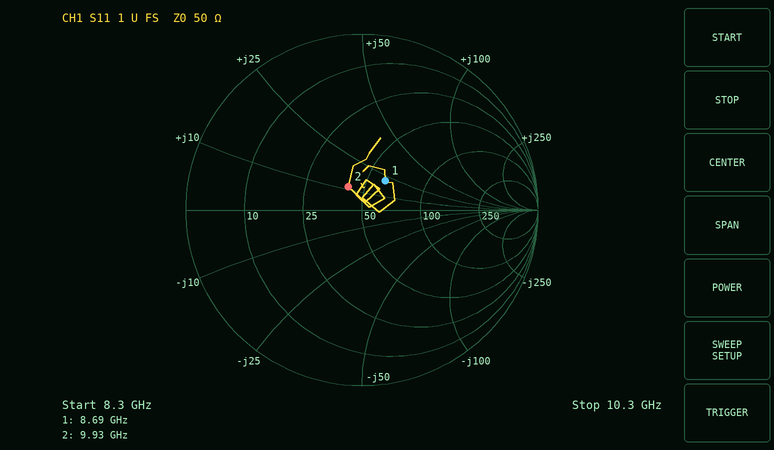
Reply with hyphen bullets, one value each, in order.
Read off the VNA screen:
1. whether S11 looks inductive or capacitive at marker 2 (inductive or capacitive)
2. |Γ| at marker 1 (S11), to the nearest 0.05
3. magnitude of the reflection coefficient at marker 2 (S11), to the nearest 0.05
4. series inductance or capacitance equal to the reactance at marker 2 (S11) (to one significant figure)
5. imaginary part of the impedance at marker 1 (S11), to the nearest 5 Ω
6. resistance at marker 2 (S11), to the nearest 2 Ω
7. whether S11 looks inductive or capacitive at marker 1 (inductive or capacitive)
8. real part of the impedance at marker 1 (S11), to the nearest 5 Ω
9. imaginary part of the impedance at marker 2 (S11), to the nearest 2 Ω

- inductive
- 0.20
- 0.15
- 200 pH
- +20 Ω
- 42 Ω
- inductive
- 60 Ω
- +12 Ω
